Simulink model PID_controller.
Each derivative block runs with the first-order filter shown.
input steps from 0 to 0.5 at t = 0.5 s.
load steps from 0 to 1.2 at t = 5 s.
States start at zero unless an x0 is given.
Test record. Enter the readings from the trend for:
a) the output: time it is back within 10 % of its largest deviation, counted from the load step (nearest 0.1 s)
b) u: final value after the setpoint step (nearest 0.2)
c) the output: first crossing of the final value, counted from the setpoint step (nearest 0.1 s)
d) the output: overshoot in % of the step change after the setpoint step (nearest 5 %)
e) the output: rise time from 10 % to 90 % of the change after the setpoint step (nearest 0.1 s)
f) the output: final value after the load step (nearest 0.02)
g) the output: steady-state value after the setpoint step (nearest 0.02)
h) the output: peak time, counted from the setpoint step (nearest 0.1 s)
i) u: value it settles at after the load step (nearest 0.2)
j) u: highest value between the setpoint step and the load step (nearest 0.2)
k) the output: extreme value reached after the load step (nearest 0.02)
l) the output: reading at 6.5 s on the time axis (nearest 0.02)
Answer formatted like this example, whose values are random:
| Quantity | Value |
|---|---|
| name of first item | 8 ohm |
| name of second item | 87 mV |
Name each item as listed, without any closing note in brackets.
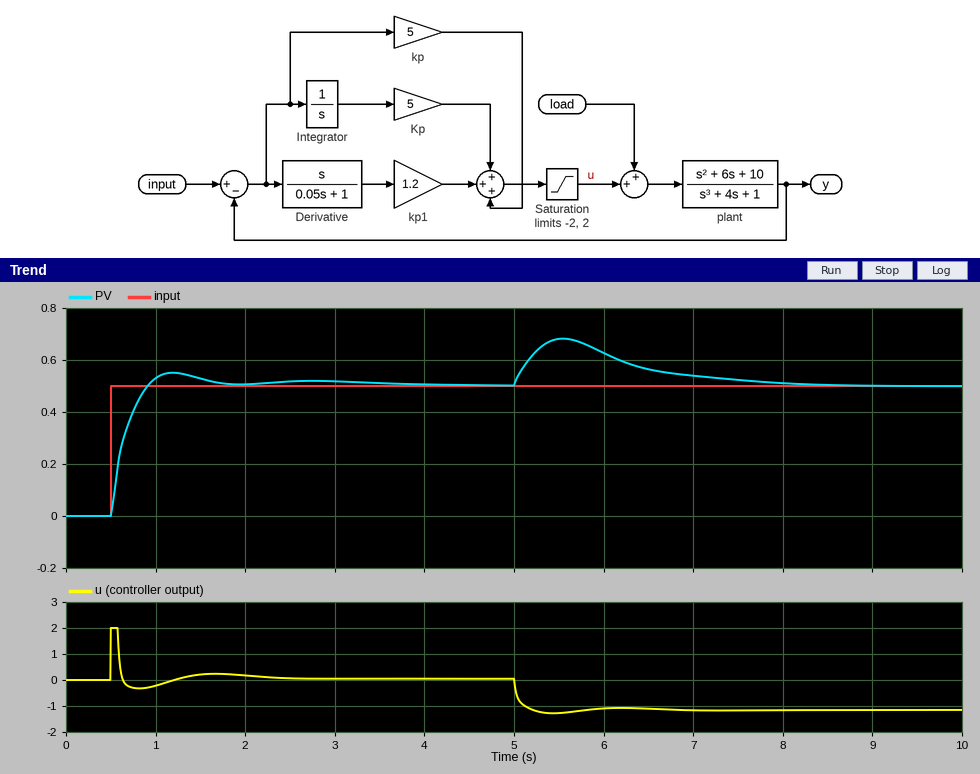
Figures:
| Quantity | Value |
|---|---|
| the output: time it is back within 10 % of its largest deviation, counted from the load step | 2.7 s |
| u: final value after the setpoint step | 0.0 |
| the output: first crossing of the final value, counted from the setpoint step | 0.4 s |
| the output: overshoot in % of the step change after the setpoint step | 10 % |
| the output: rise time from 10 % to 90 % of the change after the setpoint step | 0.3 s |
| the output: final value after the load step | 0.50 |
| the output: steady-state value after the setpoint step | 0.50 |
| the output: peak time, counted from the setpoint step | 0.7 s |
| u: value it settles at after the load step | -1.2 |
| u: highest value between the setpoint step and the load step | 2.0 |
| the output: extreme value reached after the load step | 0.68 |
| the output: reading at 6.5 s on the time axis | 0.56 |
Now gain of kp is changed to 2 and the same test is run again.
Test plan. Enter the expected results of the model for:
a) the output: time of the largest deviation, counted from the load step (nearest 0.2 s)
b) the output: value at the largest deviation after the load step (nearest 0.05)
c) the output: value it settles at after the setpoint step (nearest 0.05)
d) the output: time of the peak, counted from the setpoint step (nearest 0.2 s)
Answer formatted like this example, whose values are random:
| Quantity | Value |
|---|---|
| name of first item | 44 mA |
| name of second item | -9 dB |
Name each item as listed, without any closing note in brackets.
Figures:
| Quantity | Value |
|---|---|
| the output: time of the largest deviation, counted from the load step | 0.6 s |
| the output: value at the largest deviation after the load step | 0.80 |
| the output: value it settles at after the setpoint step | 0.50 |
| the output: time of the peak, counted from the setpoint step | 1.0 s |
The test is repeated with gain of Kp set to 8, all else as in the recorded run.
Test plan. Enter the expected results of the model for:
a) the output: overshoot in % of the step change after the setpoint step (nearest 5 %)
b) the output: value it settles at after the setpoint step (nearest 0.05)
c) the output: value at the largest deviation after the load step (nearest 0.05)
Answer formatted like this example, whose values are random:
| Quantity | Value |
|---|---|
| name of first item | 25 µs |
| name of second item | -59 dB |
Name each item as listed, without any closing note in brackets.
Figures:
| Quantity | Value |
|---|---|
| the output: overshoot in % of the step change after the setpoint step | 15 % |
| the output: value it settles at after the setpoint step | 0.50 |
| the output: value at the largest deviation after the load step | 0.65 |
